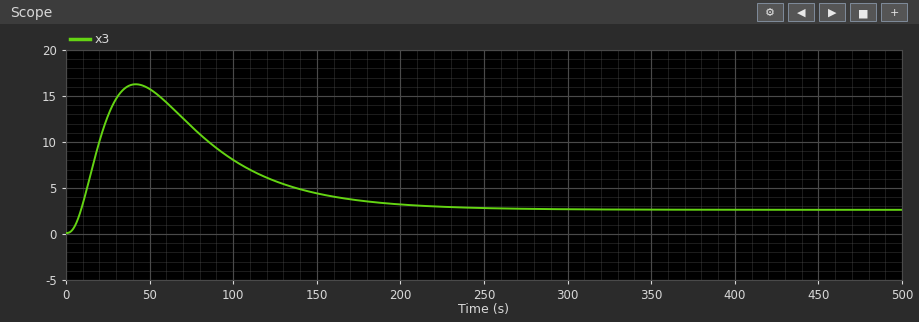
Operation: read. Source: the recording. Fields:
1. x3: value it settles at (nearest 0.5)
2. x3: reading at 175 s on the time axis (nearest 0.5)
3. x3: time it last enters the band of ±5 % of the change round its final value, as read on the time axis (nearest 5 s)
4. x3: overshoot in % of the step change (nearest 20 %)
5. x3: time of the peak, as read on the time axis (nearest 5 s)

2.5
3.5
270 s
540 %
40 s
